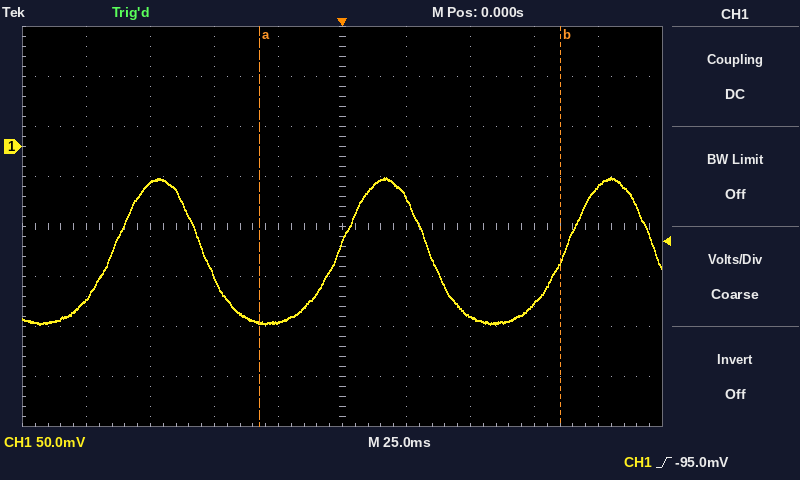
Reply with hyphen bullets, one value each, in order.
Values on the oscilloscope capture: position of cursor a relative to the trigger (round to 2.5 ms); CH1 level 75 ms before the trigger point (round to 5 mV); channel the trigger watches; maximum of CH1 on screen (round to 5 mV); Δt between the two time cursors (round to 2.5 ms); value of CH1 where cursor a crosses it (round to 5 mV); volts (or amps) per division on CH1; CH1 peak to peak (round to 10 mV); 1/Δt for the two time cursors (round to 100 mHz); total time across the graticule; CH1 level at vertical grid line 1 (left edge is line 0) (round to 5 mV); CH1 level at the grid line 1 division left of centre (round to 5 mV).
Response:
- -32.5 ms
- -35 mV
- CH1
- -30 mV
- 117.5 ms
- -175 mV
- 50 mV
- 150 mV
- 8.5 Hz
- 250 ms
- -155 mV
- -175 mV
